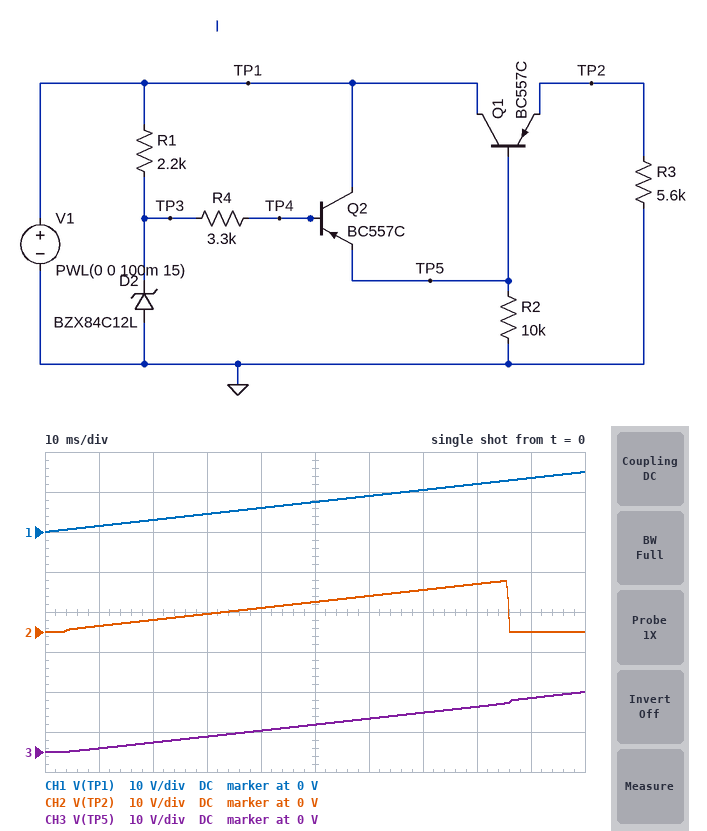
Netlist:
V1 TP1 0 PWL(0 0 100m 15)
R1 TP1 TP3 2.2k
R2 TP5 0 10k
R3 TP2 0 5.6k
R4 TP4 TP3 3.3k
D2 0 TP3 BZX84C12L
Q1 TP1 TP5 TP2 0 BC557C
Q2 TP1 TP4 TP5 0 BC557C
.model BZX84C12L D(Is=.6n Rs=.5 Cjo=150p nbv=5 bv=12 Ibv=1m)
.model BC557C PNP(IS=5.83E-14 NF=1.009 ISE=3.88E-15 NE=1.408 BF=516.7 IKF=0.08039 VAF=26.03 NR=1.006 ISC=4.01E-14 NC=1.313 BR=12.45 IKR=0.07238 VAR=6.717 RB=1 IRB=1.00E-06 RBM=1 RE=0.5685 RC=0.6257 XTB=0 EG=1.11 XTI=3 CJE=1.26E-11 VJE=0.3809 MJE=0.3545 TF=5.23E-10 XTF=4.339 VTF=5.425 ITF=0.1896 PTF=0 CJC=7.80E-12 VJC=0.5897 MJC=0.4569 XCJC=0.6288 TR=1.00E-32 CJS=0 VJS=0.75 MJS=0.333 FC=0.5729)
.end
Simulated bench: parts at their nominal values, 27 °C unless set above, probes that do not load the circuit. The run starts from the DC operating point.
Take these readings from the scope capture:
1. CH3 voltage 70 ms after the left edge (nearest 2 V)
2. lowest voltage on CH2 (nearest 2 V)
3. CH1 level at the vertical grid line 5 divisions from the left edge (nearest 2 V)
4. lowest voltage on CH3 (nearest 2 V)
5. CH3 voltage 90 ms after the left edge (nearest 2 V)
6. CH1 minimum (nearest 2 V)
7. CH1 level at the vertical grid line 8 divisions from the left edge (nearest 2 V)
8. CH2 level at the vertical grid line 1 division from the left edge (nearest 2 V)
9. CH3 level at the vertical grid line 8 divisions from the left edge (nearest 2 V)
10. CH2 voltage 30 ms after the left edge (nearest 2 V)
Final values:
10 V
0 V
8 V
0 V
14 V
0 V
12 V
2 V
12 V
4 V
